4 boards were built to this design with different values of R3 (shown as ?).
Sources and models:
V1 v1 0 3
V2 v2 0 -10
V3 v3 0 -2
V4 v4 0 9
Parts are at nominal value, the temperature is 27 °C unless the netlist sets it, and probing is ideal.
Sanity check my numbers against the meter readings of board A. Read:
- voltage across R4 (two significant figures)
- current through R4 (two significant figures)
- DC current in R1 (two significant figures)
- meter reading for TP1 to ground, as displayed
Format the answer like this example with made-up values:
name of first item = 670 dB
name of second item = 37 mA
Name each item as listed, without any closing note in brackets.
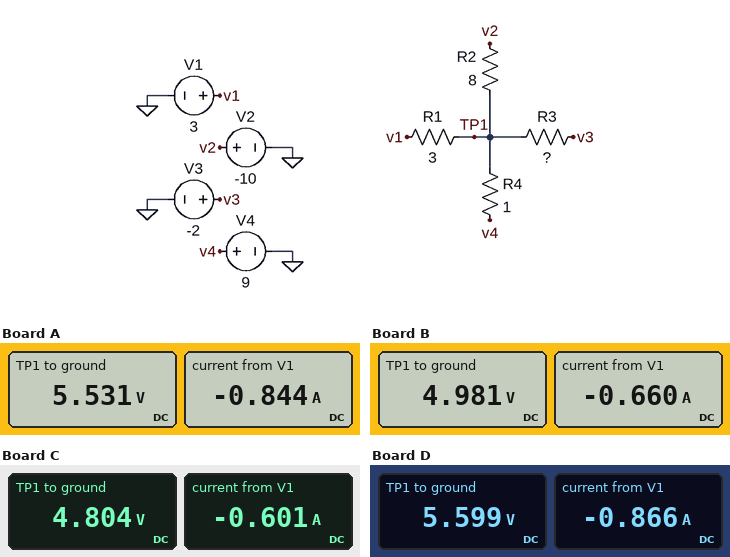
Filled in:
voltage across R4 = 3.5 V
current through R4 = 3.5 A
DC current in R1 = 840 mA
meter reading for TP1 to ground, as displayed = 5.531 V
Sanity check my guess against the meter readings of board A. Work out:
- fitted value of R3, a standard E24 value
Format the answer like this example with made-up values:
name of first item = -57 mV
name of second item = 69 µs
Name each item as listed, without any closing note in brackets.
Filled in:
fitted value of R3, a standard E24 value = 11 Ω
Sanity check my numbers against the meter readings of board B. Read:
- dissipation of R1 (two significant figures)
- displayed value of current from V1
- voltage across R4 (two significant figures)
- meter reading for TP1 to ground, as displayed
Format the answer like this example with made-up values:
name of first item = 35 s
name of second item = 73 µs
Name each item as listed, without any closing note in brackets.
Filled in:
dissipation of R1 = 1.3 W
displayed value of current from V1 = -0.660 A
voltage across R4 = 4.0 V
meter reading for TP1 to ground, as displayed = 4.981 V
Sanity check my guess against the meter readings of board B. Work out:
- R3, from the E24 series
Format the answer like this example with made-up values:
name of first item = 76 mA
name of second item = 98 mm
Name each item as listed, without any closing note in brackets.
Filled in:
R3, from the E24 series = 4.7 Ω
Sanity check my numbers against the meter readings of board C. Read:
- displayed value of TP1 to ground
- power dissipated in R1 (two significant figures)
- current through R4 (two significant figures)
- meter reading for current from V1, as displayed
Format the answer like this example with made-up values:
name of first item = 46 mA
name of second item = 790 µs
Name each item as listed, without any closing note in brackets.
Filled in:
displayed value of TP1 to ground = 4.804 V
power dissipated in R1 = 1.1 W
current through R4 = 4.2 A
meter reading for current from V1, as displayed = -0.601 A
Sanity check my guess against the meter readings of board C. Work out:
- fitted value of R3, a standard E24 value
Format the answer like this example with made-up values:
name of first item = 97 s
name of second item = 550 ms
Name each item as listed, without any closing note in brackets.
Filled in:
fitted value of R3, a standard E24 value = 3.9 Ω
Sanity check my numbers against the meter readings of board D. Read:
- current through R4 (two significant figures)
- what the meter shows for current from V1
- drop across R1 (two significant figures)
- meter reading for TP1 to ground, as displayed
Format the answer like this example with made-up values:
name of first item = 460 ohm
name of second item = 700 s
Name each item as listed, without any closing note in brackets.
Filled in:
current through R4 = 3.4 A
what the meter shows for current from V1 = -0.866 A
drop across R1 = 2.6 V
meter reading for TP1 to ground, as displayed = 5.599 V
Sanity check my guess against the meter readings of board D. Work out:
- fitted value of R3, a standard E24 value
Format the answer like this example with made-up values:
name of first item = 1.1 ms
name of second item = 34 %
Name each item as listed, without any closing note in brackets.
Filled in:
fitted value of R3, a standard E24 value = 13 Ω
